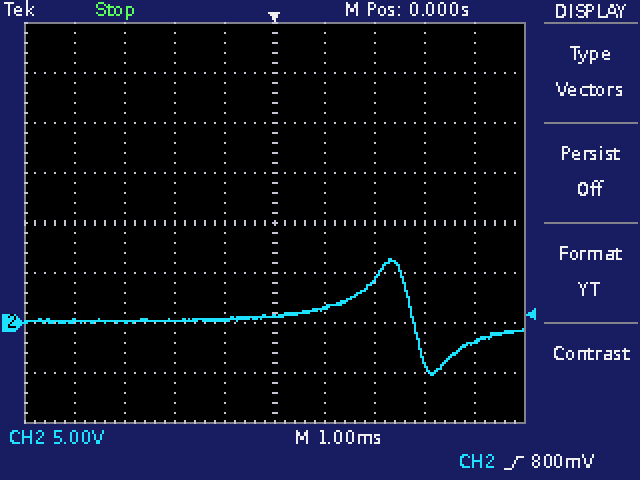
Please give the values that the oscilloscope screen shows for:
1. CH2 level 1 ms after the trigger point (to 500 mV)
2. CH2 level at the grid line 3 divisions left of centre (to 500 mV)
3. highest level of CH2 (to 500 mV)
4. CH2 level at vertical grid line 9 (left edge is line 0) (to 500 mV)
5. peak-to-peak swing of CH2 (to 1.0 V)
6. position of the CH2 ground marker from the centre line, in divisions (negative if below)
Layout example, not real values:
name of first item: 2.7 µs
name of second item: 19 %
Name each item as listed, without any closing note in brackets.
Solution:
CH2 level 1 ms after the trigger point: 1.5 V
CH2 level at the grid line 3 divisions left of centre: 0.0 V
highest level of CH2: 6.5 V
CH2 level at vertical grid line 9 (left edge is line 0): -2.0 V
peak-to-peak swing of CH2: 12.0 V
position of the CH2 ground marker from the centre line, in divisions: -2.0 div
